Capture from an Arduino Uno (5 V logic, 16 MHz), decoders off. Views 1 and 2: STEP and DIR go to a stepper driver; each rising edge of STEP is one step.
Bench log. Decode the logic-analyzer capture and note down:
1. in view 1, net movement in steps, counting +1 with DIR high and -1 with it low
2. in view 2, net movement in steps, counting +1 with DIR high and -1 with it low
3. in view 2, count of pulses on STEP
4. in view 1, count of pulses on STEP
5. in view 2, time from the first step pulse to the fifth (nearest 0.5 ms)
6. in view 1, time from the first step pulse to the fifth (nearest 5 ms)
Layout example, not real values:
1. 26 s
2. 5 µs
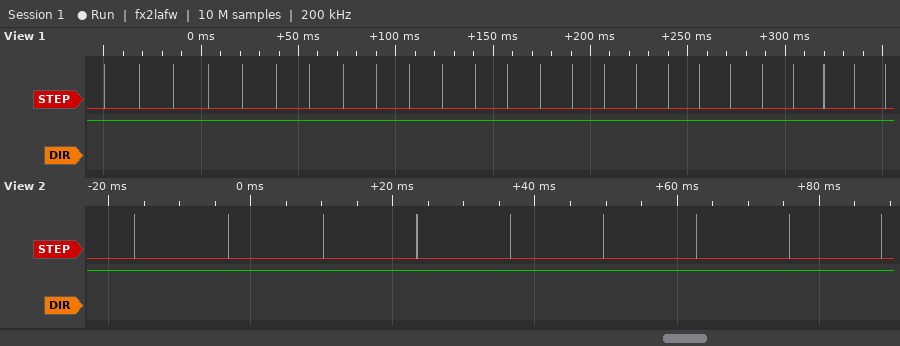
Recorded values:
1. +25
2. +9
3. 9
4. 25
5. 53.0 ms
6. 70 ms
